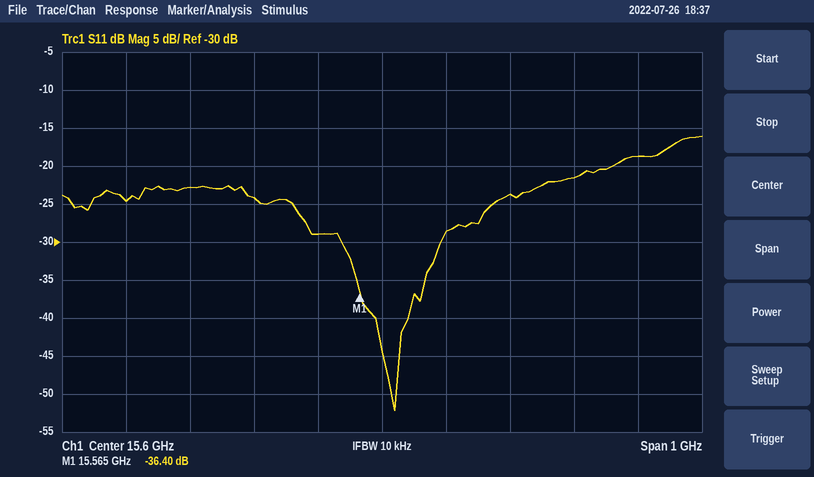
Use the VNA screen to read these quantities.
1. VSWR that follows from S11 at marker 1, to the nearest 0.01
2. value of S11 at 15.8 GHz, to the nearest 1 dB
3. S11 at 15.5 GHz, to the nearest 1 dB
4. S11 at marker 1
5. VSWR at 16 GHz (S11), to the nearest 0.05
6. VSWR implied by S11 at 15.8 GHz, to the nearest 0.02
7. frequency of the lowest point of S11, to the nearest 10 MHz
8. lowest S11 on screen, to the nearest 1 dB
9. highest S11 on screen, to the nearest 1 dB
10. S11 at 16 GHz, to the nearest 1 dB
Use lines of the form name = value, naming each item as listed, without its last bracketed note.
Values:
VSWR that follows from S11 at marker 1, to the nearest 0.01 = 1.03
value of S11 at 15.8 GHz, to the nearest 1 dB = -24 dB
S11 at 15.5 GHz, to the nearest 1 dB = -29 dB
S11 at marker 1 = -36.40 dB
VSWR at 16 GHz (S11), to the nearest 0.05 = 1.25
VSWR implied by S11 at 15.8 GHz, to the nearest 0.02 = 1.14
frequency of the lowest point of S11, to the nearest 10 MHz = 15.62 GHz
lowest S11 on screen, to the nearest 1 dB = -52 dB
highest S11 on screen, to the nearest 1 dB = -16 dB
S11 at 16 GHz, to the nearest 1 dB = -19 dB
